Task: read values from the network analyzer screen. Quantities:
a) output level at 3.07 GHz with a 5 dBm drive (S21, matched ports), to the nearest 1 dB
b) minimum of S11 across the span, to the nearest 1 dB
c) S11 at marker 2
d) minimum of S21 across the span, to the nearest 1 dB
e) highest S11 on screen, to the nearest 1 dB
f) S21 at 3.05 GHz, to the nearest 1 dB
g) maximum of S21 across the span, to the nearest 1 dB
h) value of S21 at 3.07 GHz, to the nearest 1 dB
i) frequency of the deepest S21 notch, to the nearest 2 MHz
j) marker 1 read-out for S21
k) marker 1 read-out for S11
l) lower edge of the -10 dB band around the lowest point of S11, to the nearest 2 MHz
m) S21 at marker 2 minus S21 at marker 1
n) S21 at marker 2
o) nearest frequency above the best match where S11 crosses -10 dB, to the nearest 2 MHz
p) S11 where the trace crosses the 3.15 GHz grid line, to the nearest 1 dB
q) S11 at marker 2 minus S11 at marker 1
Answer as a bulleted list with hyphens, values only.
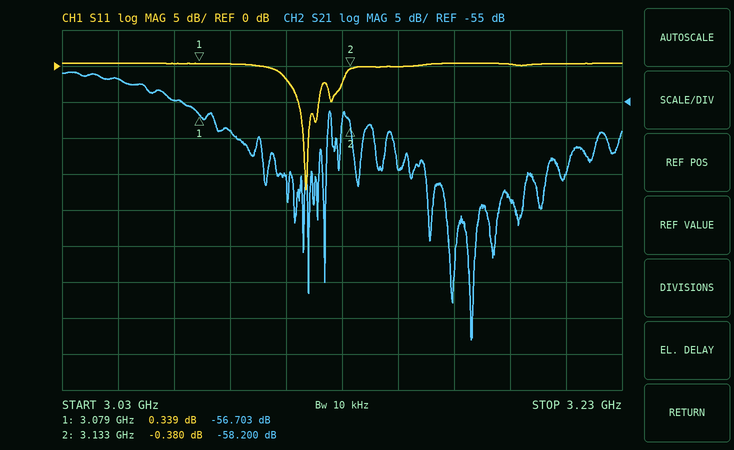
- -50 dBm
- -17 dB
- -0.380 dB
- -88 dB
- 0 dB
- -52 dB
- -51 dB
- -55 dB
- 3.176 GHz
- -56.703 dB
- 0.339 dB
- 3.116 GHz
- -1.497 dB
- -58.200 dB
- 3.118 GHz
- 0 dB
- -0.719 dB
